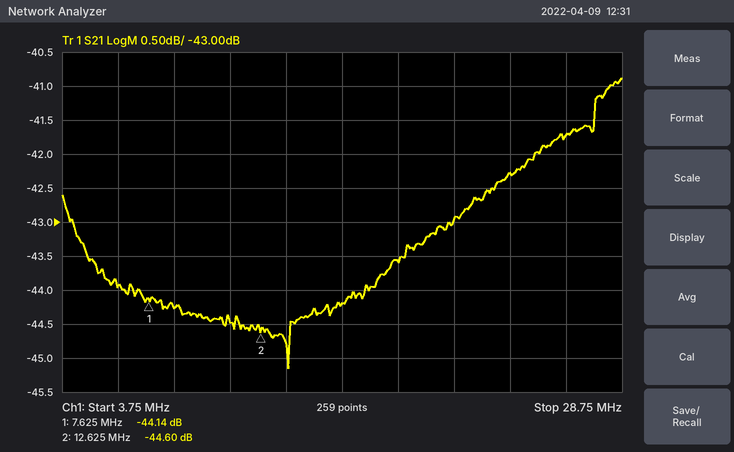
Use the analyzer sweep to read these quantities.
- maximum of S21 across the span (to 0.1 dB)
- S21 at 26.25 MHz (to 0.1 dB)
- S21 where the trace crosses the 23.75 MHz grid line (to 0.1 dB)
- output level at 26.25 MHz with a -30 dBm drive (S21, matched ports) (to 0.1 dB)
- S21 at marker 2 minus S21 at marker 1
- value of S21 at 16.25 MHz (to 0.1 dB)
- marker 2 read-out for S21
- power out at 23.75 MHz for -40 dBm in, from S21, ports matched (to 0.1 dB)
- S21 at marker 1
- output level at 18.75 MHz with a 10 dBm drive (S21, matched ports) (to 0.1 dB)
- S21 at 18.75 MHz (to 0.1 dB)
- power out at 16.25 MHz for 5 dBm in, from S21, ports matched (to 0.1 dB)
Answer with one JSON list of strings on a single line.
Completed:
["-40.9 dB", "-41.7 dB", "-42.3 dB", "-71.7 dBm", "-0.46 dB", "-44.2 dB", "-44.60 dB", "-82.3 dBm", "-44.14 dB", "-33.6 dBm", "-43.6 dB", "-39.2 dBm"]
